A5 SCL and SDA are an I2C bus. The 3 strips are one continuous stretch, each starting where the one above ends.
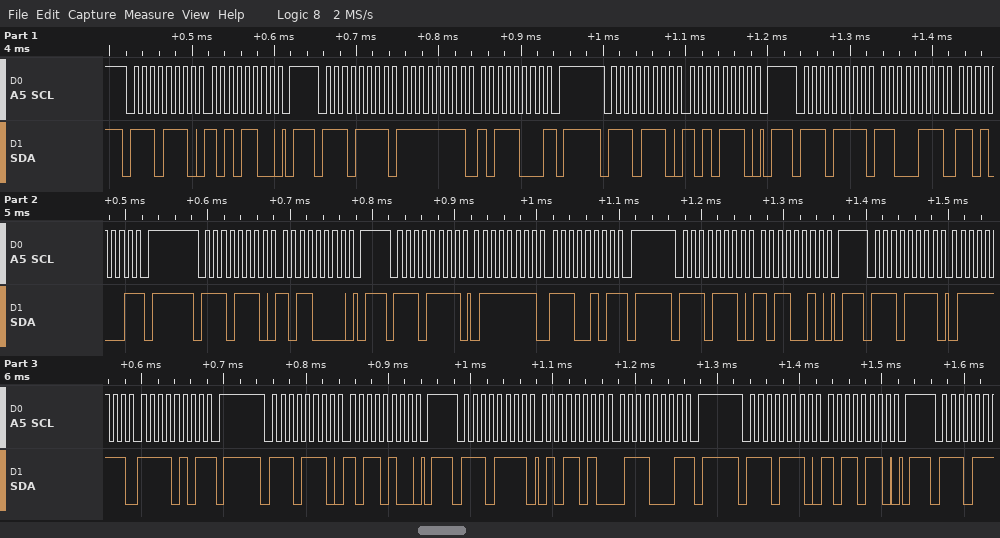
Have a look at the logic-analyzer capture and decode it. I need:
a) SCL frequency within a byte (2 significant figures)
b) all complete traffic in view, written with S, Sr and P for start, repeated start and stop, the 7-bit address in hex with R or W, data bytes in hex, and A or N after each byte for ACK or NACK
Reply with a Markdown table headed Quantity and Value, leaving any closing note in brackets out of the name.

| Quantity | Value |
|---|---|
| SCL frequency within a byte | 100 kHz |
| all complete traffic in view, written with S, Sr and P for start, repeated start and stop, the 7-bit address in hex with R or W, data bytes in hex, and A or N after each byte for ACK or NACK | S 77W A AC A P S 77R A FF A B8 N P S 77W A AE A P S 77R A C7 A D1 N P S 77W A B0 A P S 77R A 7F A E5 N P S 77W A B2 A P S 77R A 7F A F5 N P S 77W A B4 A P S 77R A 5A A 71 N P S 77W A B6 A P |
